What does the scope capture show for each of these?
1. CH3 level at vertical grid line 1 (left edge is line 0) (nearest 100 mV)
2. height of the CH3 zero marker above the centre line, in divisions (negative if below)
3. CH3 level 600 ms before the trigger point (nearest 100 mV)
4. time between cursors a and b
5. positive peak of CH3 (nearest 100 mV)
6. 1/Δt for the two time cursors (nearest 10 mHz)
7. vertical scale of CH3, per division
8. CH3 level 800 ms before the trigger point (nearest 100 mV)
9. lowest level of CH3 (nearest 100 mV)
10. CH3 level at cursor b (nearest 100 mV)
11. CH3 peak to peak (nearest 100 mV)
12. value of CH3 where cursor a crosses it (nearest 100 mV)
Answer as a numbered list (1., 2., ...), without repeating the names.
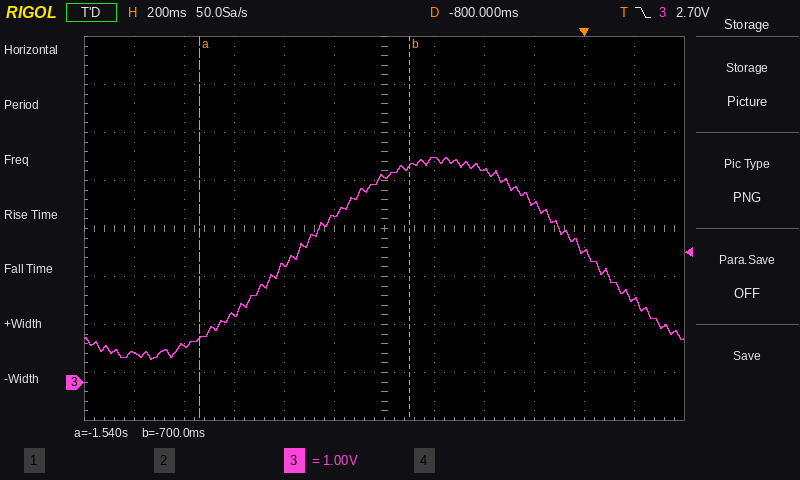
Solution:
1. 600 mV
2. -3.2 div
3. 4.7 V
4. 840 ms
5. 4.7 V
6. 1.19 Hz
7. 1 V
8. 4.3 V
9. 500 mV
10. 4.5 V
11. 4.2 V
12. 900 mV
